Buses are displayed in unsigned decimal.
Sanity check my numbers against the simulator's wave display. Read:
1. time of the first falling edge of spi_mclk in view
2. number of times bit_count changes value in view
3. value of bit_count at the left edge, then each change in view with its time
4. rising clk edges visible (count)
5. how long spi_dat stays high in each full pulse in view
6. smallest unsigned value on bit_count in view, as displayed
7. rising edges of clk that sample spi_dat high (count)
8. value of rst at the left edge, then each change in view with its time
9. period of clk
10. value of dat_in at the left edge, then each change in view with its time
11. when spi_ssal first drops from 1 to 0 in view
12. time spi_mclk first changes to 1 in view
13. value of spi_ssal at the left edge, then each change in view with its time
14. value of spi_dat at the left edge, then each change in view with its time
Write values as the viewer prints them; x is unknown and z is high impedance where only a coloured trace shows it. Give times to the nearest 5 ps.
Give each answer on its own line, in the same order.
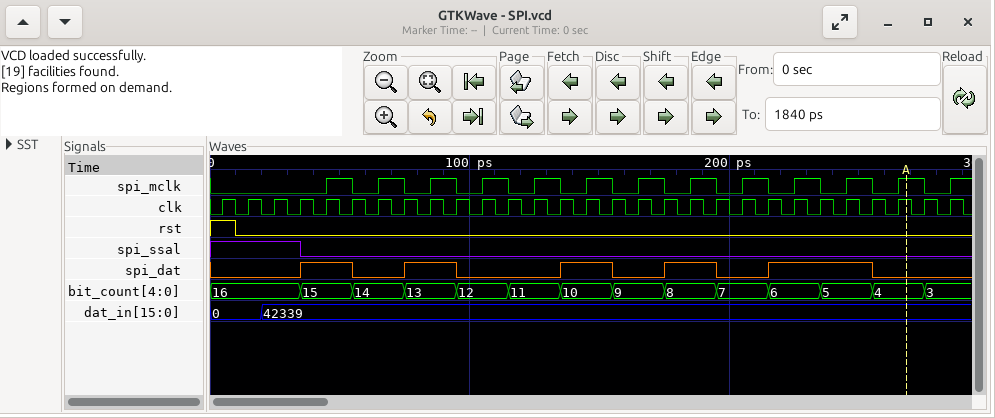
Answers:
55 ps
13
16, 15 at 35 ps, 14 at 55 ps, 13 at 75 ps, 12 at 95 ps, 11 at 115 ps, 10 at 135 ps, 9 at 155 ps, 8 at 175 ps, 7 at 195 ps, 6 at 215 ps, 5 at 235 ps, 4 at 255 ps, 3 at 275 ps
29
20 ps, 20 ps, 20 ps, 20 ps, 40 ps
3
12
1, 0 at 10 ps
10 ps
0, 42339 at 20 ps
35 ps
45 ps
1, 0 at 35 ps
0, 1 at 35 ps, 0 at 55 ps, 1 at 75 ps, 0 at 95 ps, 1 at 135 ps, 0 at 155 ps, 1 at 175 ps, 0 at 195 ps, 1 at 215 ps, 0 at 255 ps
